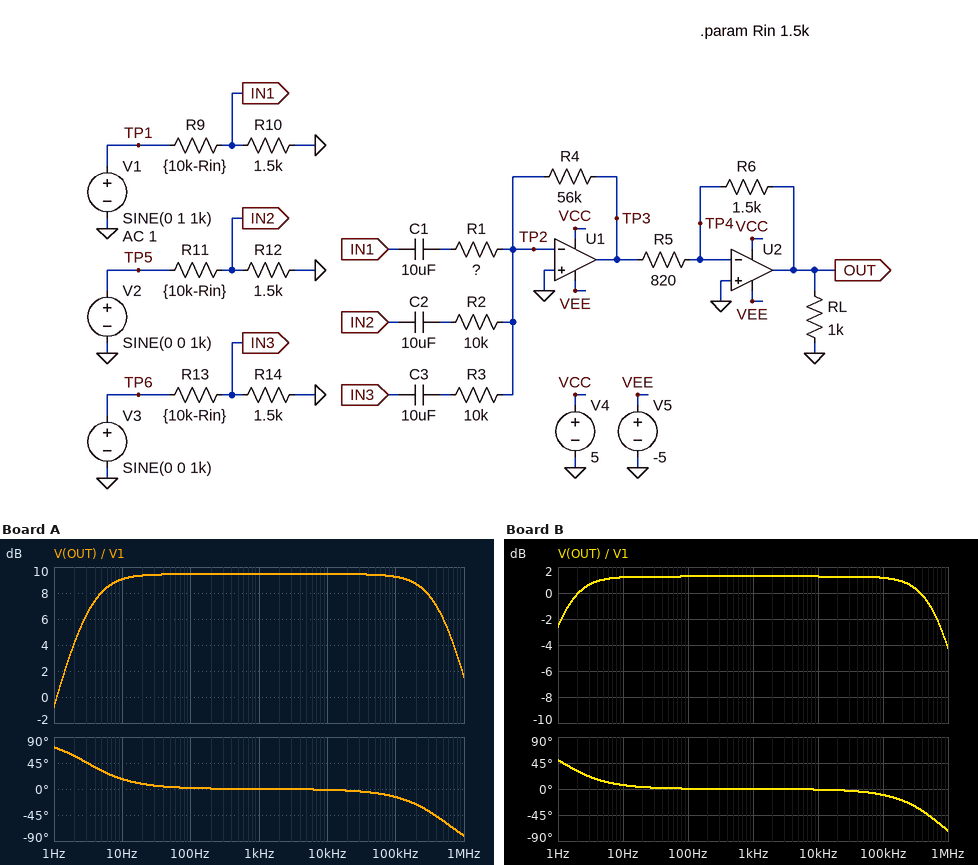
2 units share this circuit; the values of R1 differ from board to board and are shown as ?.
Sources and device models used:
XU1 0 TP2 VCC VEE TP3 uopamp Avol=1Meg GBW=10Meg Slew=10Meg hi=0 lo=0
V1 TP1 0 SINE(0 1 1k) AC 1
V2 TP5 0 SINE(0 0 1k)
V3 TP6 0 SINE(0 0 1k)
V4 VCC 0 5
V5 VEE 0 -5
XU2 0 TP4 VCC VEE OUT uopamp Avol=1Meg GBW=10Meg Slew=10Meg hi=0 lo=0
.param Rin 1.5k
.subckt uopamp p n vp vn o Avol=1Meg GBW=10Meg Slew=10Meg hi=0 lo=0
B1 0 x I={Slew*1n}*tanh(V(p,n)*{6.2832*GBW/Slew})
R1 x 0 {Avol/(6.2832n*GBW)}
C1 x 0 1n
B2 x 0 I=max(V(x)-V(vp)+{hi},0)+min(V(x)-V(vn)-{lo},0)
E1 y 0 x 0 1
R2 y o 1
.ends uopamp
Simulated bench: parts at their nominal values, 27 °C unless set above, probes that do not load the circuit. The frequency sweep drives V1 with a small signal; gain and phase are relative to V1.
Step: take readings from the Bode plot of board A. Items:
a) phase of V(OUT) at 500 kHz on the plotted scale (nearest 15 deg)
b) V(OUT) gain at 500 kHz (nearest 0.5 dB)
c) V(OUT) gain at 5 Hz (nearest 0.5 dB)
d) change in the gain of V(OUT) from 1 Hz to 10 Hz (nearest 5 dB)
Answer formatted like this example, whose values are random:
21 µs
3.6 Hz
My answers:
-60 deg
6.0 dB
8.0 dB
10 dB
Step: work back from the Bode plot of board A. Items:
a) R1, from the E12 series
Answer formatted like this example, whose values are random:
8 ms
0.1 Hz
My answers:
3.9 kΩ
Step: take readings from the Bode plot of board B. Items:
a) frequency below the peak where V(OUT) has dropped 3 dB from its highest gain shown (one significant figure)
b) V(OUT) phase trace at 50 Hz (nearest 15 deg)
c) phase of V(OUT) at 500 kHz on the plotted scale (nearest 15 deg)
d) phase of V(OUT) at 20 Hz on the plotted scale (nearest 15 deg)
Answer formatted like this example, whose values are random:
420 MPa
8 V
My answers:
1 Hz
0 deg
-45 deg
0 deg
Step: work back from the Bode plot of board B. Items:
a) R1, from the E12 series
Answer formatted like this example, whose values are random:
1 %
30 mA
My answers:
12 kΩ
